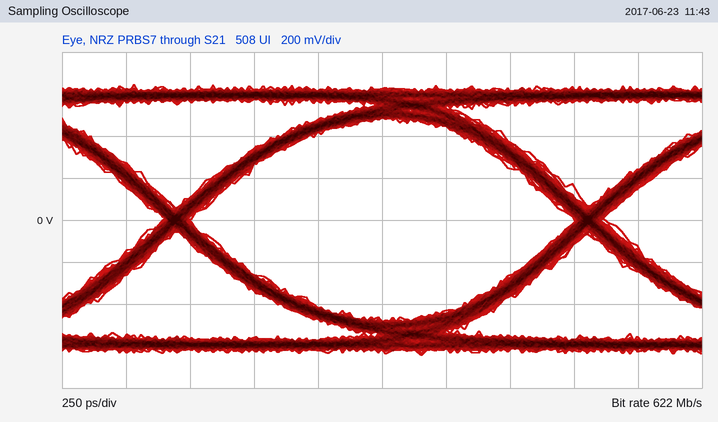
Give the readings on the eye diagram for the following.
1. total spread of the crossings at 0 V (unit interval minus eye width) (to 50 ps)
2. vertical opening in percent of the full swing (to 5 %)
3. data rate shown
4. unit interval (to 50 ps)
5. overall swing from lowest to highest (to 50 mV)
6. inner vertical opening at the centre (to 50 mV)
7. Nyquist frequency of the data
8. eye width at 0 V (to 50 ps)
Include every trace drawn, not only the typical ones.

100 ps
75 %
622 Mb/s
1.60 ns
1.30 V
950 mV
311 MHz
1.50 ns
